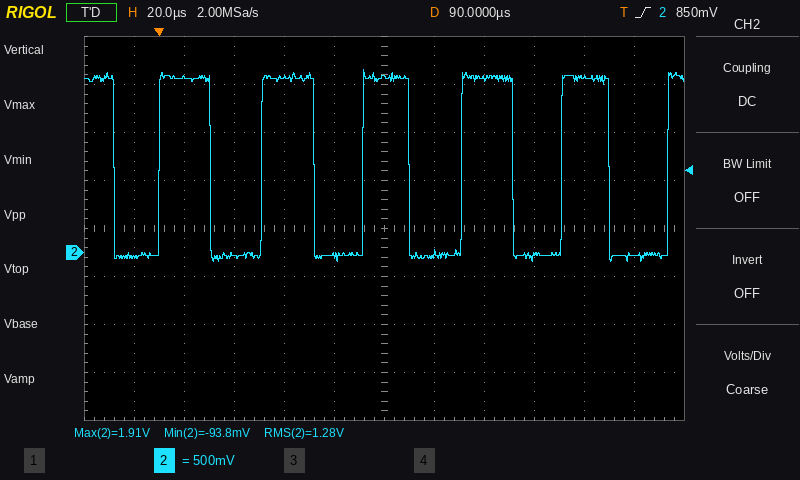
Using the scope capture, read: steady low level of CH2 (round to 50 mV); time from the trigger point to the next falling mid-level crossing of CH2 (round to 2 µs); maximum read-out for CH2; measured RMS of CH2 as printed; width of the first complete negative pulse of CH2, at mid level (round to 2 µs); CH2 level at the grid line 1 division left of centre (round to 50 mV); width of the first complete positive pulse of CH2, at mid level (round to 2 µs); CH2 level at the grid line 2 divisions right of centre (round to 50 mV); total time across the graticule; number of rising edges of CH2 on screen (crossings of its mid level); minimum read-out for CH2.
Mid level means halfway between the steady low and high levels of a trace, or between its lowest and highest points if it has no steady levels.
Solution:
-50 mV
20 µs
1.91 V
1.28 V
18 µs
-50 mV
20 µs
1.80 V
240 µs
6
-93.8 mV
